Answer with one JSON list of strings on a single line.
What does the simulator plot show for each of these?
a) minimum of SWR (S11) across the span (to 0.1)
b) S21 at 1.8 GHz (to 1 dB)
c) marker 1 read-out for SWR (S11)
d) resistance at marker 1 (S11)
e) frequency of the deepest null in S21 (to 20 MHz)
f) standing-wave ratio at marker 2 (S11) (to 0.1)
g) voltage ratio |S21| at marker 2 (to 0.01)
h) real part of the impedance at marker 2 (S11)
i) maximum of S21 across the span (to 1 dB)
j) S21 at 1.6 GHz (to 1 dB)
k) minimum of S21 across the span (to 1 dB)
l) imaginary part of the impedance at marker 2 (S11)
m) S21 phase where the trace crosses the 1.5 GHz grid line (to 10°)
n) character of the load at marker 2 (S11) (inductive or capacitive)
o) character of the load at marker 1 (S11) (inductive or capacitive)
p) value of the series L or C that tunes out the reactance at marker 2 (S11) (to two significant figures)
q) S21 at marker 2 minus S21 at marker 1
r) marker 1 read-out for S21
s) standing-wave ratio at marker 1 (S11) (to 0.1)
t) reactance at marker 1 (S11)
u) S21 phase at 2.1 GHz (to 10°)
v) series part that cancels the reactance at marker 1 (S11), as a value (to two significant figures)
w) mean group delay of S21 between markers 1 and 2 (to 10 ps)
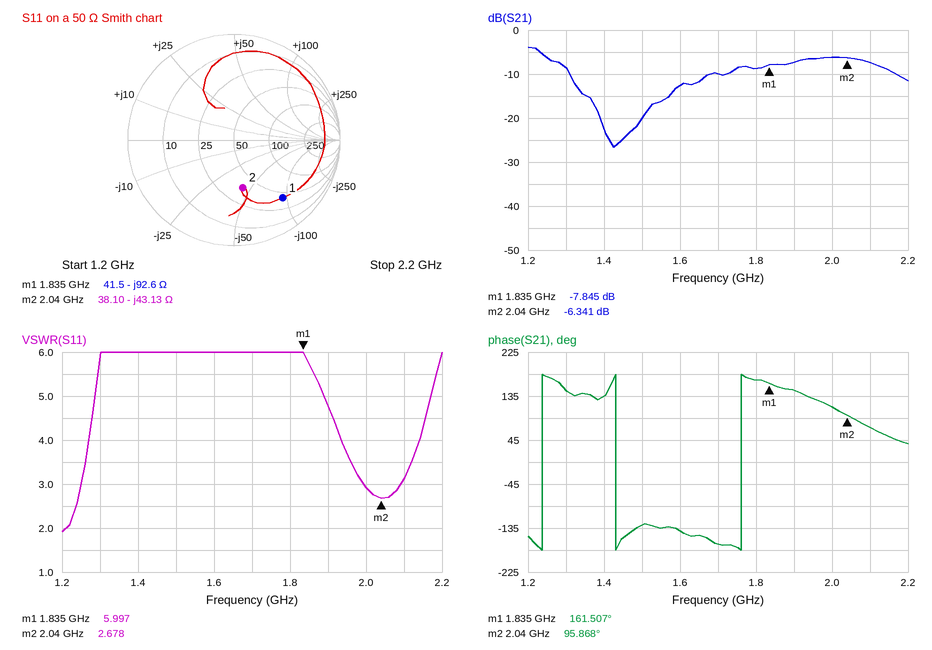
["1.9", "-9 dB", "5.997", "41.5 Ω", "1.42 GHz", "2.7", "0.48", "38.10 Ω", "-4 dB", "-13 dB", "-27 dB", "-43.13 Ω", "-130°", "capacitive", "capacitive", "3.4 nH", "1.504 dB", "-7.845 dB", "6.0", "-92.6 Ω", "70°", "8.0 nH", "890 ps"]
